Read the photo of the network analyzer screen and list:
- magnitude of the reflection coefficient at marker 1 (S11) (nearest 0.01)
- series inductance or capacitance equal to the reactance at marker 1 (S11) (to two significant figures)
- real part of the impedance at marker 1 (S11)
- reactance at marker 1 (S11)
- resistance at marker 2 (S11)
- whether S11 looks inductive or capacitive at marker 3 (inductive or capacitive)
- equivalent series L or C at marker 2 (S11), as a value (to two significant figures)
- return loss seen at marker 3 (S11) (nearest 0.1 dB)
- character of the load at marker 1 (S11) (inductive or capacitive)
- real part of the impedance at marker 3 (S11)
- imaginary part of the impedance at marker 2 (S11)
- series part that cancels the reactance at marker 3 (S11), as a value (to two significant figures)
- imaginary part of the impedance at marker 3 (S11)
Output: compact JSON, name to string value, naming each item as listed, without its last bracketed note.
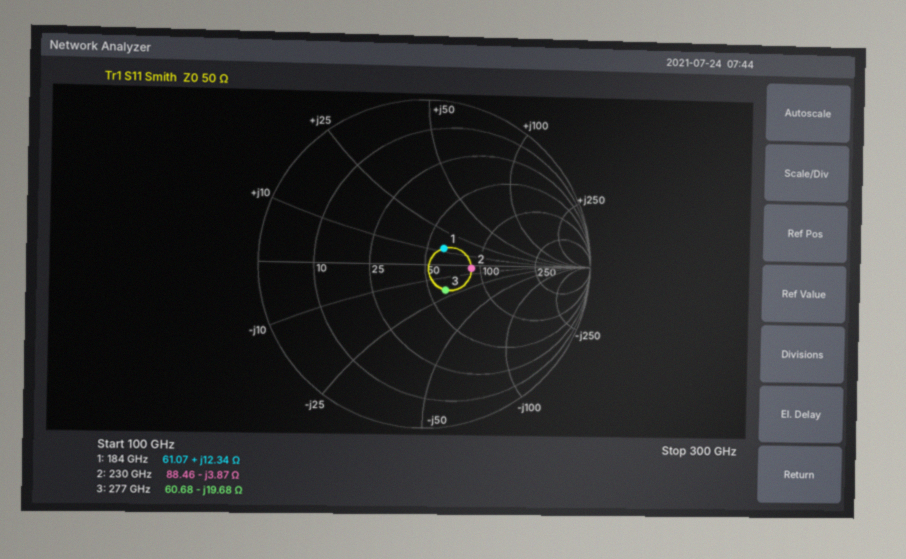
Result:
{"magnitude of the reflection coefficient at marker 1 (S11)": "0.15", "series inductance or capacitance equal to the reactance at marker 1 (S11)": "11 pH", "real part of the impedance at marker 1": "61.07 Ω", "reactance at marker 1": "+12.34 Ω", "resistance at marker 2": "88.46 Ω", "whether S11 looks inductive or capacitive at marker 3": "capacitive", "equivalent series L or C at marker 2 (S11), as a value": "180 fF", "return loss seen at marker 3 (S11)": "14.0 dB", "character of the load at marker 1 (S11)": "inductive", "real part of the impedance at marker 3": "60.68 Ω", "imaginary part of the impedance at marker 2": "-3.87 Ω", "series part that cancels the reactance at marker 3 (S11), as a value": "11 pH", "imaginary part of the impedance at marker 3": "-19.68 Ω"}
